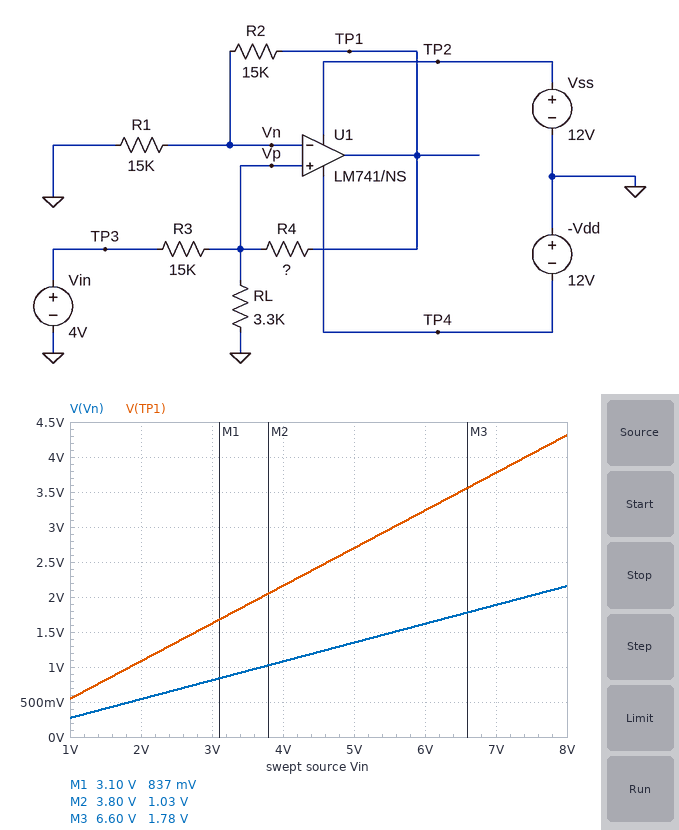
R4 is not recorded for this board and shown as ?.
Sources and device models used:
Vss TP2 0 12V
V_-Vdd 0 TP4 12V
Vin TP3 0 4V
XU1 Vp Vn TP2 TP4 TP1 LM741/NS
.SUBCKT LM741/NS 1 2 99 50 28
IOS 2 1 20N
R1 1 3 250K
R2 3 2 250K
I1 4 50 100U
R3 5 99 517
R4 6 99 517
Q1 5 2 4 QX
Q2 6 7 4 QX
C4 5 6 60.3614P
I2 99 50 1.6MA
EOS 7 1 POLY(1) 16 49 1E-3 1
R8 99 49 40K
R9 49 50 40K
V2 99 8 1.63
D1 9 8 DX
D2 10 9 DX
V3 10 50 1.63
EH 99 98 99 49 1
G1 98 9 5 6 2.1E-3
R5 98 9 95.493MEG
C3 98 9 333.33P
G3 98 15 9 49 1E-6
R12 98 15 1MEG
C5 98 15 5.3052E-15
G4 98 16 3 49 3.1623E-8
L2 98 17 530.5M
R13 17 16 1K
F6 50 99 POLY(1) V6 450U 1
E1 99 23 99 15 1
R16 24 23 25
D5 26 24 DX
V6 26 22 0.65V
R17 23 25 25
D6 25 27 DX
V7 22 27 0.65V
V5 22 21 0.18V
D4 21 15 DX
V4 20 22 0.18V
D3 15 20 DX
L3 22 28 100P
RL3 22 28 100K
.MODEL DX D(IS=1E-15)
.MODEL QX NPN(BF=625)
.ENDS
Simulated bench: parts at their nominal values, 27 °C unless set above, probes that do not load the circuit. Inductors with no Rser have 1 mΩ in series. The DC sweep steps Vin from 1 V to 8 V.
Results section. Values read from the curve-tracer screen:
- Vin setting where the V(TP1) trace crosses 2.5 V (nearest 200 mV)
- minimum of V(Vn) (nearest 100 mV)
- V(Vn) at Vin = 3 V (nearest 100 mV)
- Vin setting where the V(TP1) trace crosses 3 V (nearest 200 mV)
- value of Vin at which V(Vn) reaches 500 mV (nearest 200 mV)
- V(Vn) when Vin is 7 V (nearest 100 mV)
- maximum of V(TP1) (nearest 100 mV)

4.6 V
300 mV
800 mV
5.6 V
1.8 V
1.9 V
4.3 V
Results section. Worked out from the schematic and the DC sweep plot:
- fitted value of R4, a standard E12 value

8.2 kΩ
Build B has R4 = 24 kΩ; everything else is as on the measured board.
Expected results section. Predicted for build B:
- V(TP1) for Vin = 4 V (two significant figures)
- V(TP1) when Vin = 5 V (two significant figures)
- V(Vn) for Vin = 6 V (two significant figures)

1.6 V
2.0 V
1.2 V
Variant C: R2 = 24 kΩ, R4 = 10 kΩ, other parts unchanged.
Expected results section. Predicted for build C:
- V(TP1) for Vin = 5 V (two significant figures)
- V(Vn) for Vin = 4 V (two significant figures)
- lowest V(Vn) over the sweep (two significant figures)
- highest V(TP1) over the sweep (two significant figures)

4.1 V
1.3 V
320 mV
6.6 V
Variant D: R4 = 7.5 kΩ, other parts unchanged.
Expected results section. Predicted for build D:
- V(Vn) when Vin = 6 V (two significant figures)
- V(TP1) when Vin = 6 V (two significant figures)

1.7 V
3.4 V
